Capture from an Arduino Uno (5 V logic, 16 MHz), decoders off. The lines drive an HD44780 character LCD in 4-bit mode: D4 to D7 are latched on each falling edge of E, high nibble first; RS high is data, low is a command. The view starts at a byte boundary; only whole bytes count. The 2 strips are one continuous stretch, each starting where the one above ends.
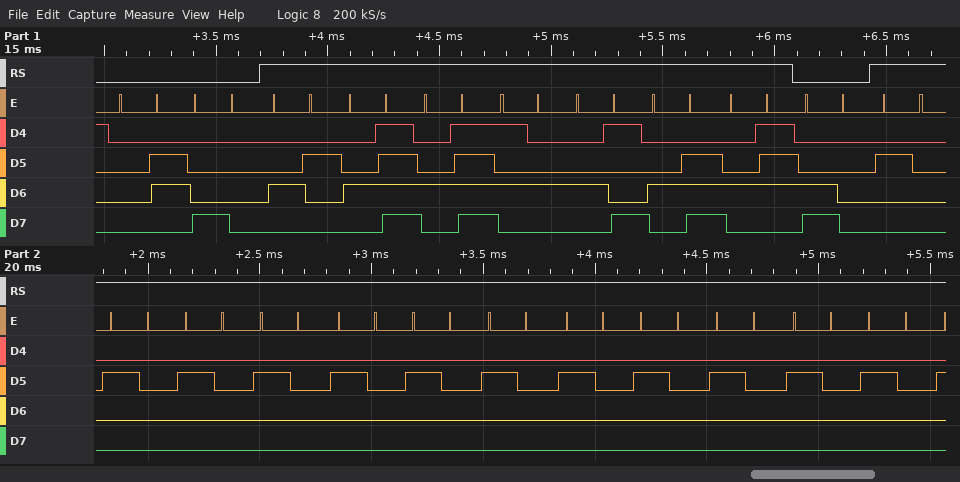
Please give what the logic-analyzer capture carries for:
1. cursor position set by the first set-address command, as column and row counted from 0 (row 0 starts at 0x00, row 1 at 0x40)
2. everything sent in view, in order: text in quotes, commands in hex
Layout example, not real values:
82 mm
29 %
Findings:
column 0, row 0
0x06 0x80 "BOOTING" 0xC0 "            "
